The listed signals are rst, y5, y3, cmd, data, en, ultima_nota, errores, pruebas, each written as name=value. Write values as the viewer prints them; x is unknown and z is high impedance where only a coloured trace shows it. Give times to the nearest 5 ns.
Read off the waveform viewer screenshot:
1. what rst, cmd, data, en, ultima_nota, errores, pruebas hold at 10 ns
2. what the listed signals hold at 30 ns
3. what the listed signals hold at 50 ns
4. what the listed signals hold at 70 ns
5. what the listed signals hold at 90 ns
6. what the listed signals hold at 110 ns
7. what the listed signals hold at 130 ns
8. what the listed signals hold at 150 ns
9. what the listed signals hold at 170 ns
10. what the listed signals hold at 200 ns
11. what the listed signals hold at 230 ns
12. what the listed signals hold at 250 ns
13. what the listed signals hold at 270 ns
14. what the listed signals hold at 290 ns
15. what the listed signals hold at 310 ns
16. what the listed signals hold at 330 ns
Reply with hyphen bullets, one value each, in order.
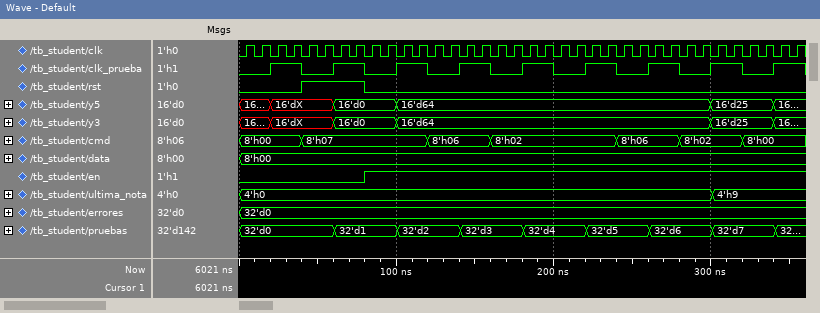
- rst=0, cmd=8'h00, data=8'h00, en=0, ultima_nota=4'h0, errores=32'd0, pruebas=32'd0
- rst=0, y5=16'dX, y3=16'dX, cmd=8'h00, data=8'h00, en=0, ultima_nota=4'h0, errores=32'd0, pruebas=32'd0
- rst=1, y5=16'dX, y3=16'dX, cmd=8'h07, data=8'h00, en=0, ultima_nota=4'h0, errores=32'd0, pruebas=32'd0
- rst=1, y5=16'd0, y3=16'd0, cmd=8'h07, data=8'h00, en=0, ultima_nota=4'h0, errores=32'd0, pruebas=32'd1
- rst=0, y5=16'd0, y3=16'd0, cmd=8'h07, data=8'h00, en=1, ultima_nota=4'h0, errores=32'd0, pruebas=32'd1
- rst=0, y5=16'd64, y3=16'd64, cmd=8'h07, data=8'h00, en=1, ultima_nota=4'h0, errores=32'd0, pruebas=32'd2
- rst=0, y5=16'd64, y3=16'd64, cmd=8'h06, data=8'h00, en=1, ultima_nota=4'h0, errores=32'd0, pruebas=32'd2
- rst=0, y5=16'd64, y3=16'd64, cmd=8'h06, data=8'h00, en=1, ultima_nota=4'h0, errores=32'd0, pruebas=32'd3
- rst=0, y5=16'd64, y3=16'd64, cmd=8'h02, data=8'h00, en=1, ultima_nota=4'h0, errores=32'd0, pruebas=32'd3
- rst=0, y5=16'd64, y3=16'd64, cmd=8'h02, data=8'h00, en=1, ultima_nota=4'h0, errores=32'd0, pruebas=32'd4
- rst=0, y5=16'd64, y3=16'd64, cmd=8'h02, data=8'h00, en=1, ultima_nota=4'h0, errores=32'd0, pruebas=32'd5
- rst=0, y5=16'd64, y3=16'd64, cmd=8'h06, data=8'h00, en=1, ultima_nota=4'h0, errores=32'd0, pruebas=32'd5
- rst=0, y5=16'd64, y3=16'd64, cmd=8'h06, data=8'h00, en=1, ultima_nota=4'h0, errores=32'd0, pruebas=32'd6
- rst=0, y5=16'd64, y3=16'd64, cmd=8'h02, data=8'h00, en=1, ultima_nota=4'h0, errores=32'd0, pruebas=32'd6
- rst=0, y5=16'd25, y3=16'd25, cmd=8'h02, data=8'h00, en=1, ultima_nota=4'h9, errores=32'd0, pruebas=32'd7
- rst=0, y5=16'd25, y3=16'd25, cmd=8'h00, data=8'h00, en=1, ultima_nota=4'h9, errores=32'd0, pruebas=32'd7
